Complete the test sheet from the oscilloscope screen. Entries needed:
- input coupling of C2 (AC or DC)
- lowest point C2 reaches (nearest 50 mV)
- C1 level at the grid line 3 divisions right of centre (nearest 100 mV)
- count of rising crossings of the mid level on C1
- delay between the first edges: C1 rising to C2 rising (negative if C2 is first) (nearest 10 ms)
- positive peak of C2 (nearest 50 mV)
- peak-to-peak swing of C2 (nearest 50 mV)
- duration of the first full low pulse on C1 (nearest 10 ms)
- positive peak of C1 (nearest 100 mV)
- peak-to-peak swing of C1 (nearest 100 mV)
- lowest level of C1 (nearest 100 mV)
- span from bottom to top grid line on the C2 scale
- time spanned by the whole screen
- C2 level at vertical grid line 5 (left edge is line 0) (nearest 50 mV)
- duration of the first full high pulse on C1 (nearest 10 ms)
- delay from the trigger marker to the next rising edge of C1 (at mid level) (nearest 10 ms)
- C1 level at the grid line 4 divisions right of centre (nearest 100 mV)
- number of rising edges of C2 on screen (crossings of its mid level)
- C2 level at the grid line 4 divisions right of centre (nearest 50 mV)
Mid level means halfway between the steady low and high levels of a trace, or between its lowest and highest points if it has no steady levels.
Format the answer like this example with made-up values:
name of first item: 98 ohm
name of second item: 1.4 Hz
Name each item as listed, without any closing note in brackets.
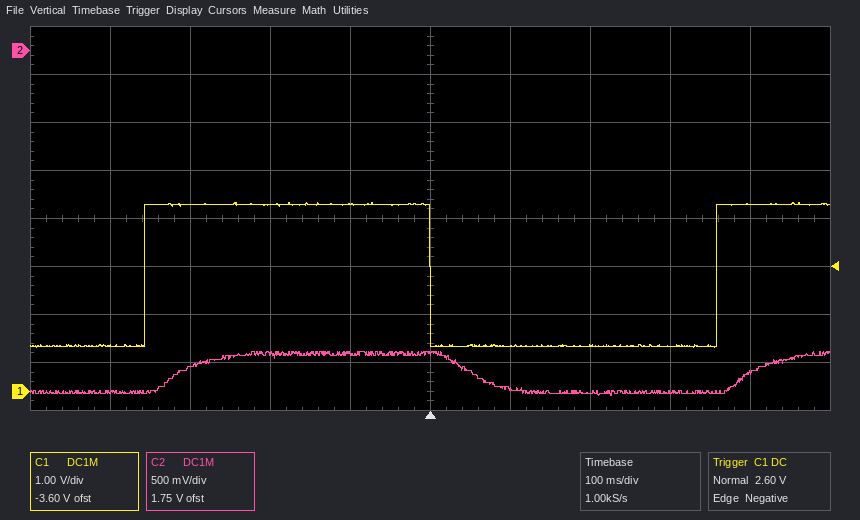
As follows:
input coupling of C2: DC
lowest point C2 reaches: -3.60 V
C1 level at the grid line 3 divisions right of centre: 900 mV
count of rising crossings of the mid level on C1: 2
delay between the first edges: C1 rising to C2 rising (negative if C2 is first): +40 ms
positive peak of C2: -3.15 V
peak-to-peak swing of C2: 450 mV
duration of the first full low pulse on C1: 360 ms
positive peak of C1: 3.9 V
peak-to-peak swing of C1: 3.0 V
lowest level of C1: 900 mV
span from bottom to top grid line on the C2 scale: 4 V
time spanned by the whole screen: 1 s
C2 level at vertical grid line 5 (left edge is line 0): -3.15 V
duration of the first full high pulse on C1: 360 ms
delay from the trigger marker to the next rising edge of C1 (at mid level): 360 ms
C1 level at the grid line 4 divisions right of centre: 3.9 V
number of rising edges of C2 on screen: 2
C2 level at the grid line 4 divisions right of centre: -3.35 V
